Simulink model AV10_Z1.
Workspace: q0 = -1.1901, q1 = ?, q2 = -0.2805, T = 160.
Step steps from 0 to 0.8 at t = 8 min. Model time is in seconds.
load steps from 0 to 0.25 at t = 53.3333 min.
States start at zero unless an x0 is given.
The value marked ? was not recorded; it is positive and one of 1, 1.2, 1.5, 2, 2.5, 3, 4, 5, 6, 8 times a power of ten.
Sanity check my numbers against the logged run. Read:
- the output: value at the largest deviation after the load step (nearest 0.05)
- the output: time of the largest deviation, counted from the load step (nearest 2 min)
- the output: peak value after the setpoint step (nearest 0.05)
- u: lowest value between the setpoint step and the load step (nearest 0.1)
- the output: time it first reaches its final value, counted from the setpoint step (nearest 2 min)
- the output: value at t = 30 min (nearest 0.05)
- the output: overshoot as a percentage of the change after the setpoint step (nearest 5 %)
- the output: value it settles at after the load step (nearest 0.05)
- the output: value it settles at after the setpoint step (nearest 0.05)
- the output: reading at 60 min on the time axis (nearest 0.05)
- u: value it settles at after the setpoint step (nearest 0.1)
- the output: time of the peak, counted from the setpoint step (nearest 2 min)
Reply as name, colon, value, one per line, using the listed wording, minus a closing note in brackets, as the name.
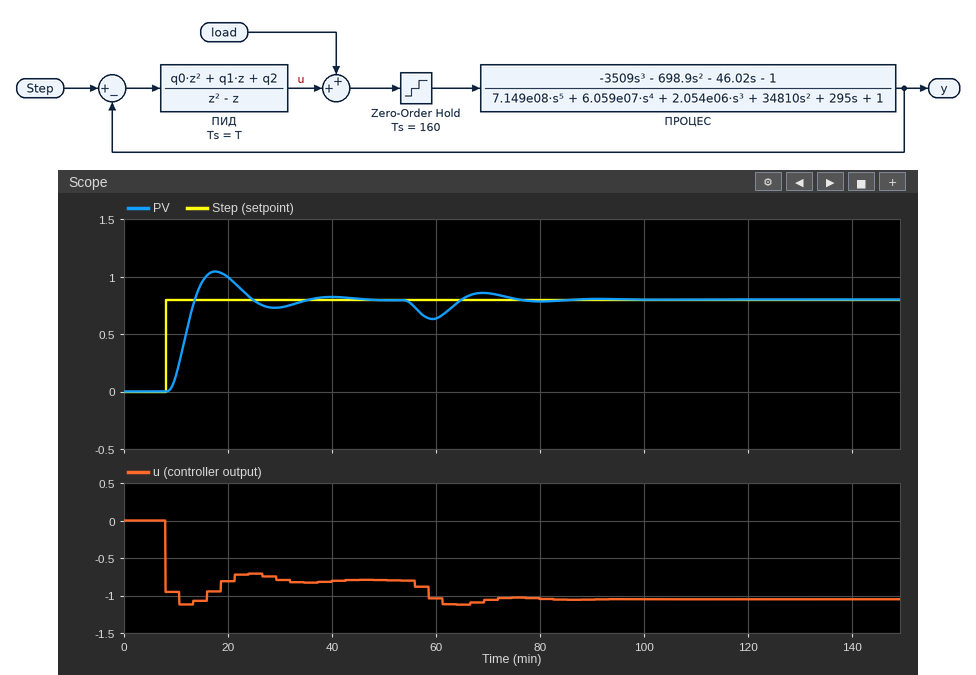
the output: value at the largest deviation after the load step: 0.65
the output: time of the largest deviation, counted from the load step: 6 min
the output: peak value after the setpoint step: 1.05
u: lowest value between the setpoint step and the load step: -1.1
the output: time it first reaches its final value, counted from the setpoint step: 6 min
the output: value at t = 30 min: 0.75
the output: overshoot as a percentage of the change after the setpoint step: 30 %
the output: value it settles at after the load step: 0.80
the output: value it settles at after the setpoint step: 0.80
the output: reading at 60 min on the time axis: 0.65
u: value it settles at after the setpoint step: -0.8
the output: time of the peak, counted from the setpoint step: 10 min
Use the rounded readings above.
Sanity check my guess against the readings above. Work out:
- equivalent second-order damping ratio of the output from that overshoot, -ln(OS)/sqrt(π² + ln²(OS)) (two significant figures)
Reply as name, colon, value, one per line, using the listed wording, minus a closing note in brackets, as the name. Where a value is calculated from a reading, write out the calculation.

equivalent second-order damping ratio of the output from that overshoot, -ln(OS)/sqrt(π² + ln²(OS)): ln(0.3) = -1.204; 1.204 / sqrt(9.870 + 1.450) = 0.36
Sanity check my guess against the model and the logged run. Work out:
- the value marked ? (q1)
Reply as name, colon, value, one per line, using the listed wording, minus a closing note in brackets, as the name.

the value marked ?: 0.6
